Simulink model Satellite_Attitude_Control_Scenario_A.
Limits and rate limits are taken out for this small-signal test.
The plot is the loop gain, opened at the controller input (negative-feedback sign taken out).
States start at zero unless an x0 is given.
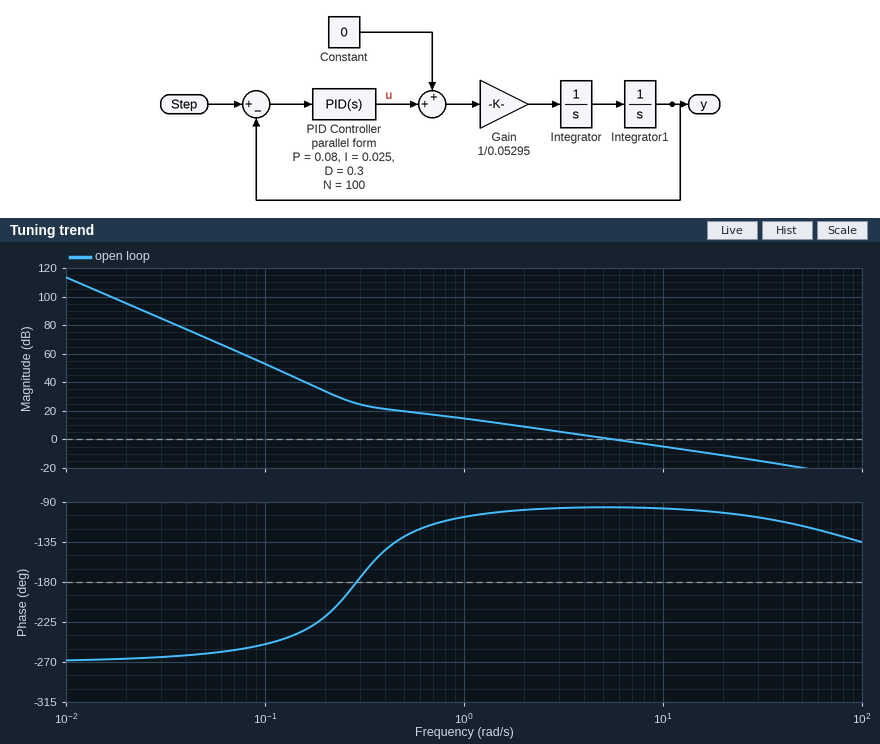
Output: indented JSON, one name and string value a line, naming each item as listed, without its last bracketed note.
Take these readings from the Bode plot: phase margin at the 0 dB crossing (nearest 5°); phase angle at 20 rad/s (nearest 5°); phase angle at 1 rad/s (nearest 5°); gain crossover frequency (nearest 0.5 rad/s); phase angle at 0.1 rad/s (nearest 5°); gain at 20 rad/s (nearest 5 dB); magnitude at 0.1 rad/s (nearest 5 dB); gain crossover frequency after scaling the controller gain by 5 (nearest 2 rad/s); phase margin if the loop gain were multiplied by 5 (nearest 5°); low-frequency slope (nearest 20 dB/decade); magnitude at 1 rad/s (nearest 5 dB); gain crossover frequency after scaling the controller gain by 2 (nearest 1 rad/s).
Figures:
{
  "phase margin at the 0 dB crossing": "85°",
  "phase angle at 20 rad/s": "-100°",
  "phase angle at 1 rad/s": "-105°",
  "gain crossover frequency": "5.5 rad/s",
  "phase angle at 0.1 rad/s": "-250°",
  "gain at 20 rad/s": "-10 dB",
  "magnitude at 0.1 rad/s": "55 dB",
  "gain crossover frequency after scaling the controller gain by 5": "28 rad/s",
  "phase margin if the loop gain were multiplied by 5": "75°",
  "low-frequency slope": "-60 dB/decade",
  "magnitude at 1 rad/s": "15 dB",
  "gain crossover frequency after scaling the controller gain by 2": "11 rad/s"
}
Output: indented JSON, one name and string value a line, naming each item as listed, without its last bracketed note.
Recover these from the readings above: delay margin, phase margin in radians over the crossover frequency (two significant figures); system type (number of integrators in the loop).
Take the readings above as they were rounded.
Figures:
{
  "delay margin, phase margin in radians over the crossover frequency": "0.27 s",
  "system type": "3"
}
